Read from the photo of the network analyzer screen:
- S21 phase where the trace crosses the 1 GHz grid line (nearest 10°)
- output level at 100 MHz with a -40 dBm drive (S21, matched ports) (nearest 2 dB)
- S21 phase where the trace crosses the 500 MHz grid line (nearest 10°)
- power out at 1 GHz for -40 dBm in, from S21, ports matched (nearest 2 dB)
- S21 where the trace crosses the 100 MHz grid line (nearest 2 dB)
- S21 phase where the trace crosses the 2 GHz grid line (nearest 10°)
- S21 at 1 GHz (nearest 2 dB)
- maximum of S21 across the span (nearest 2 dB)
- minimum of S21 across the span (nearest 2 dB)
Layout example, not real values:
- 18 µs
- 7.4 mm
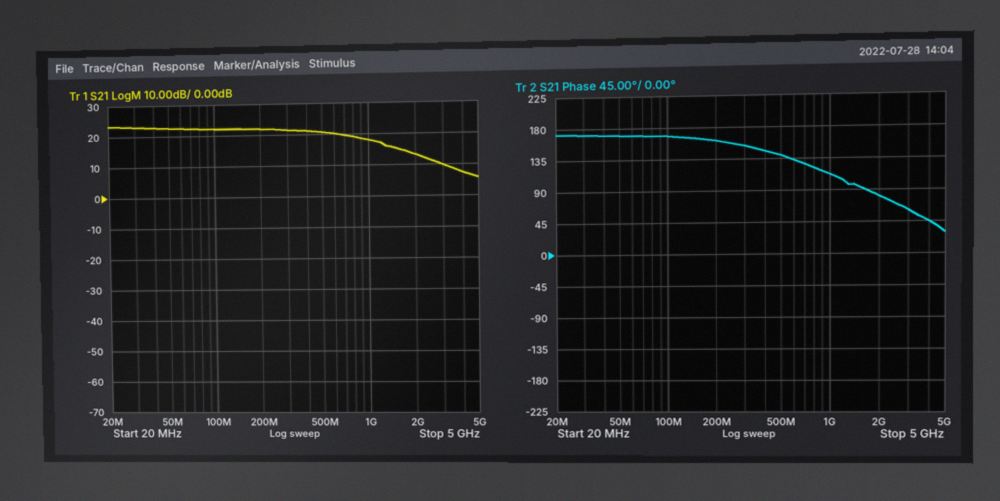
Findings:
- 110°
- -18 dBm
- 140°
- -22 dBm
- 22 dB
- 80°
- 18 dB
- 24 dB
- 6 dB
